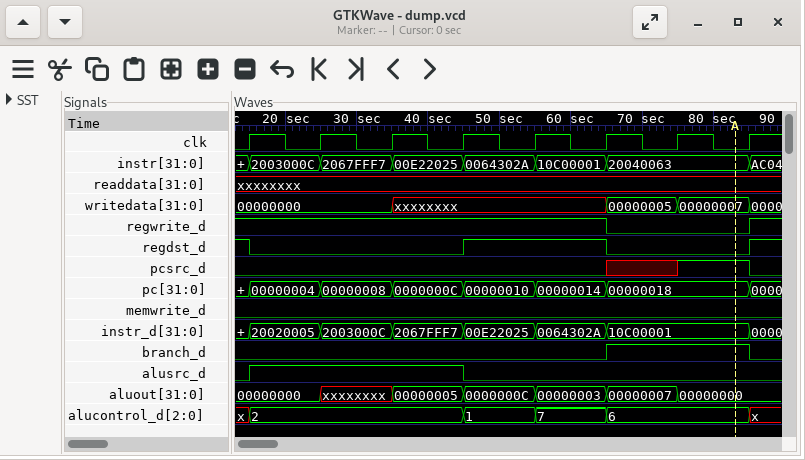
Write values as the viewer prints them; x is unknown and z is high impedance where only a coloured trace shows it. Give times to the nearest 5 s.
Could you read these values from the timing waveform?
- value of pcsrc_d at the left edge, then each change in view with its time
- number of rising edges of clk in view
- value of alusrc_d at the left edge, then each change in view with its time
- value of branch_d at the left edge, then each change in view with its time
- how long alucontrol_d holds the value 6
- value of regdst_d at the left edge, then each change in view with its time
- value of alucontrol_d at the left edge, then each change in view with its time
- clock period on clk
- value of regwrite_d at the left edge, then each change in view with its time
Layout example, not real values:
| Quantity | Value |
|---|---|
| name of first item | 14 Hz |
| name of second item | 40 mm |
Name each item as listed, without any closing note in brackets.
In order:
| Quantity | Value |
|---|---|
| value of pcsrc_d at the left edge, then each change in view with its time | 0, x at 65 s, 1 at 75 s, 0 at 85 s |
| number of rising edges of clk in view | 8 |
| value of alusrc_d at the left edge, then each change in view with its time | 0, 1 at 15 s, 0 at 45 s |
| value of branch_d at the left edge, then each change in view with its time | 0, 1 at 65 s, 0 at 85 s |
| how long alucontrol_d holds the value 6 | 20 s |
| value of regdst_d at the left edge, then each change in view with its time | 1, 0 at 15 s, 1 at 45 s, 0 at 65 s, 1 at 85 s |
| value of alucontrol_d at the left edge, then each change in view with its time | x, 2 at 15 s, 1 at 45 s, 7 at 55 s, 6 at 65 s, x at 85 s |
| clock period on clk | 10 s |
| value of regwrite_d at the left edge, then each change in view with its time | 1, 0 at 65 s, 1 at 85 s |
